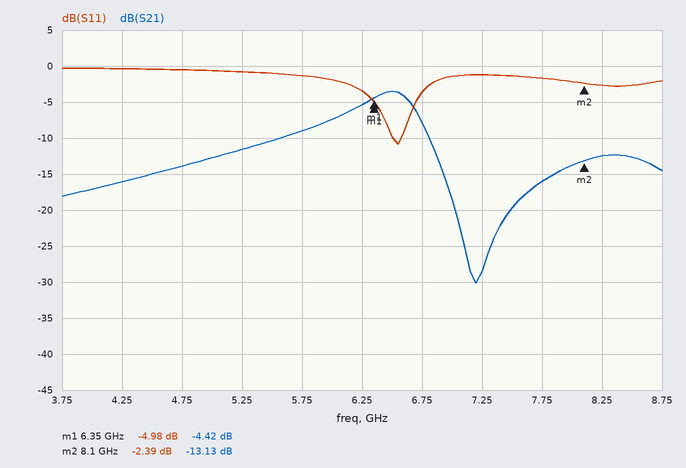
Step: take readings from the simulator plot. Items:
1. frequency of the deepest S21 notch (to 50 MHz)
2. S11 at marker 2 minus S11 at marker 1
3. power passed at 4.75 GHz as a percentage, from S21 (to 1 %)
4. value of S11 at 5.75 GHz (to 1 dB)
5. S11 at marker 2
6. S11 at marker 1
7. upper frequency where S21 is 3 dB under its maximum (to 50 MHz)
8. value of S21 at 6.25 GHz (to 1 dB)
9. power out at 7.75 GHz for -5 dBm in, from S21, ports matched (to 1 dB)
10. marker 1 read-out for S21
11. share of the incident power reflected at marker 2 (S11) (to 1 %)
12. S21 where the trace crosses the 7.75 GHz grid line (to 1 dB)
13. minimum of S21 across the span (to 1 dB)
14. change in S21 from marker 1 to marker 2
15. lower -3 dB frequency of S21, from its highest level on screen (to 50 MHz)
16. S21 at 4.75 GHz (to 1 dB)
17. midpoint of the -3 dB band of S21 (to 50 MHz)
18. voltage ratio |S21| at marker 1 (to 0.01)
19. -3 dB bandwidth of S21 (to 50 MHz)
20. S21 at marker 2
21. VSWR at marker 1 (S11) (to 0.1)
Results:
7.20 GHz
2.59 dB
4 %
-1 dB
-2.39 dB
-4.98 dB
6.70 GHz
-5 dB
-21 dBm
-4.42 dB
58 %
-16 dB
-30 dB
-8.71 dB
6.10 GHz
-14 dB
6.40 GHz
0.60
600 MHz
-13.13 dB
3.6
